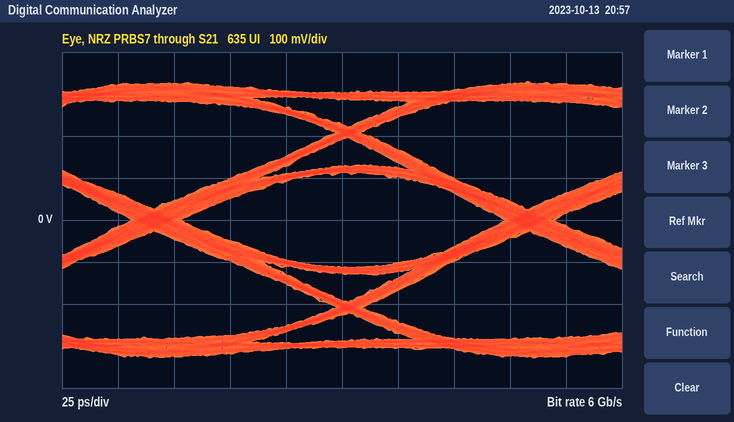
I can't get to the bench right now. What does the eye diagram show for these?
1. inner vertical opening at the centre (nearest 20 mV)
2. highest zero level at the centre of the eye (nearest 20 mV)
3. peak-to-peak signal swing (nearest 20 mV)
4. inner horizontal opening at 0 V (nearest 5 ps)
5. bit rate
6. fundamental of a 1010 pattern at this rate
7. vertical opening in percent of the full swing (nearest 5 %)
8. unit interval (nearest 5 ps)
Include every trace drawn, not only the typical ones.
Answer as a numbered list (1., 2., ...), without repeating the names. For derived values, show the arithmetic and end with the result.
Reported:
1. 220 mV
2. -120 mV
3. 660 mV
4. 145 ps
5. 6 Gb/s
6. 3 GHz
7. 220 mV / 660 mV ≈ 33.3 %, so 35 % to the nearest 5 %
8. 165 ps
